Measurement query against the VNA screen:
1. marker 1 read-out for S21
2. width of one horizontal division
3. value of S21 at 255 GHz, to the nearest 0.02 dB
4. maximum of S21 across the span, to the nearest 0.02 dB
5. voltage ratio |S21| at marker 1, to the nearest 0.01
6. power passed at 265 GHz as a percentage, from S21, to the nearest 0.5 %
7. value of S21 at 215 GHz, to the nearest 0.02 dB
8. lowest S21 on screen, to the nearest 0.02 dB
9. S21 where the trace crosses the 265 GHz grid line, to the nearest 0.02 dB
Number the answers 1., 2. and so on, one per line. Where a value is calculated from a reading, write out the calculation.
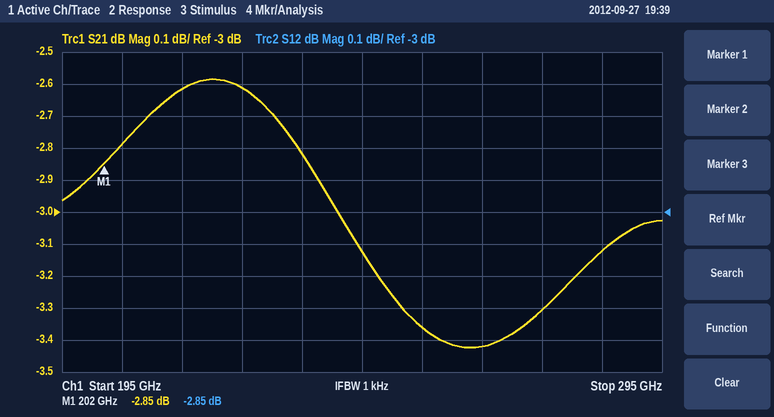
1. -2.85 dB
2. 10 GHz
3. -3.36 dB
4. -2.58 dB
5. 10^(-2.85/20) ≈ 0.72
6. 10^(-3.42/10) ≈ 45.5 %
7. -2.62 dB
8. -3.42 dB
9. -3.42 dB
